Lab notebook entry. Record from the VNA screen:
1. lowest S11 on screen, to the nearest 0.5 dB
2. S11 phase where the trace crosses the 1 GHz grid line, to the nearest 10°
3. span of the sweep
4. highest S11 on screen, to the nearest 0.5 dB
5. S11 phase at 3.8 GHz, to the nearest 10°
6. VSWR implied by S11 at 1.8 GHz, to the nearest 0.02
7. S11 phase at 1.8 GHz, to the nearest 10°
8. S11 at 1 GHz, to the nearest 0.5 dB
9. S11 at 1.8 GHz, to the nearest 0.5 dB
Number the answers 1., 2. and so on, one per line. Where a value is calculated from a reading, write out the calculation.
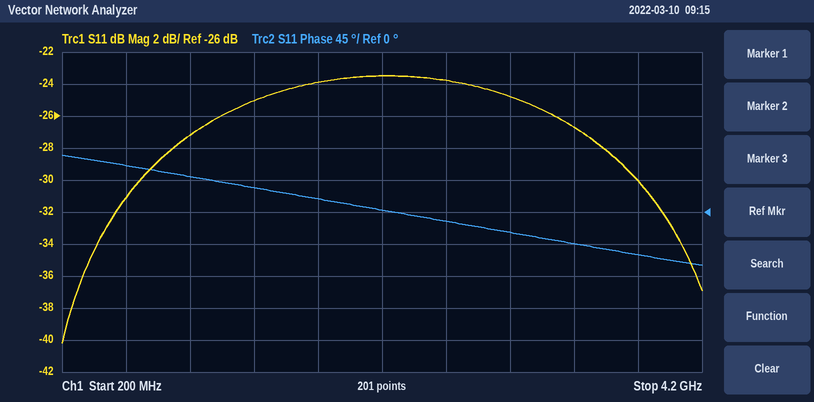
1. -40.0 dB
2. 50°
3. 4 GHz
4. -23.5 dB
5. -60°
6. |Γ| = 10^(-24/20) = 0.0631; VSWR = (1 + 0.0631)/(1 − 0.0631) ≈ 1.13, so 1.14 to the nearest 0.02
7. 20°
8. -27.0 dB
9. -24.0 dB
